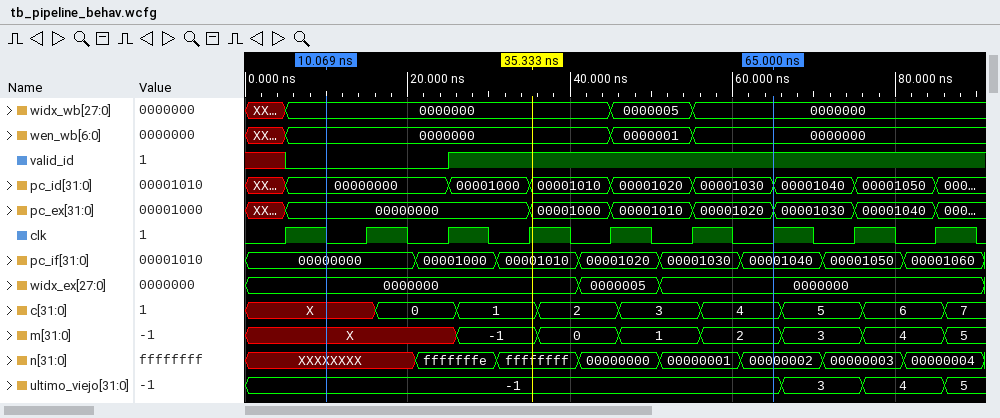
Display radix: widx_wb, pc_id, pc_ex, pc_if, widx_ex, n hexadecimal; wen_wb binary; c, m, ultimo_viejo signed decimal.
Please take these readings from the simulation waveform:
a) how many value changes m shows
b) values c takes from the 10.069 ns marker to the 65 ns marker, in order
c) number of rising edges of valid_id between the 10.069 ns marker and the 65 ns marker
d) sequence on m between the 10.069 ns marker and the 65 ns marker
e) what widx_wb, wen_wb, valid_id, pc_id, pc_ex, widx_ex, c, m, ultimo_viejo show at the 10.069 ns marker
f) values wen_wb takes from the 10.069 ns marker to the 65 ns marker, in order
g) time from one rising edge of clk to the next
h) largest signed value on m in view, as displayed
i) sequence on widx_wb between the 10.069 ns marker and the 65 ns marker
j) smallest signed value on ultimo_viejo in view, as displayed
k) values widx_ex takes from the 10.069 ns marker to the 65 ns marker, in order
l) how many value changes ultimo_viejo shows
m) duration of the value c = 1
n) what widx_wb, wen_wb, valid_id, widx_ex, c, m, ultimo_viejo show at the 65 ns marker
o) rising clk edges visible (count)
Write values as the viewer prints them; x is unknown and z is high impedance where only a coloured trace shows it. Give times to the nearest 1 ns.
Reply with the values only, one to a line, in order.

7
X, 0, 1, 2, 3, 4
1
X, -1, 0, 1, 2
widx_wb=0000000, wen_wb=0000000, valid_id=0, pc_id=00000000, pc_ex=00000000, widx_ex=0000000, c=X, m=X, ultimo_viejo=-1
0000000, 0000001, 0000000
10 ns
5
0000000, 0000005, 0000000
-1
0000000, 0000005, 0000000
3
10 ns
widx_wb=0000000, wen_wb=0000000, valid_id=1, widx_ex=0000000, c=4, m=2, ultimo_viejo=-1
9
